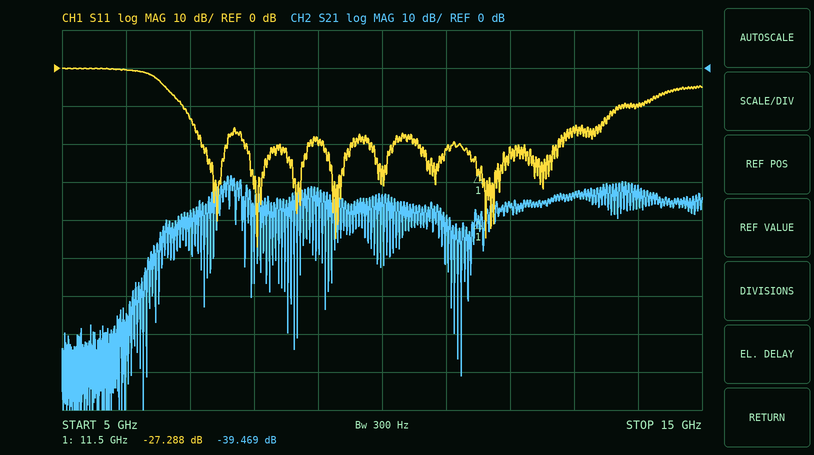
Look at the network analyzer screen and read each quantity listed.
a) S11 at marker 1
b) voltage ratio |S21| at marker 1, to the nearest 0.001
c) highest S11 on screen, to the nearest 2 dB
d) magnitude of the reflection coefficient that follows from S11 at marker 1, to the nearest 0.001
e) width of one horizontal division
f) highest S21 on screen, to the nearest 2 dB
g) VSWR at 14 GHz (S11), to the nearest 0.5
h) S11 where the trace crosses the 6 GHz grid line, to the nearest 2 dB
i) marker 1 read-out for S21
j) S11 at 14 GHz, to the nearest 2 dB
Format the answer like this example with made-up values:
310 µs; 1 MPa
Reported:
-27.288 dB; 0.011; 0 dB; 0.043; 1 GHz; -28 dB; 2.0; 0 dB; -39.469 dB; -10 dB
